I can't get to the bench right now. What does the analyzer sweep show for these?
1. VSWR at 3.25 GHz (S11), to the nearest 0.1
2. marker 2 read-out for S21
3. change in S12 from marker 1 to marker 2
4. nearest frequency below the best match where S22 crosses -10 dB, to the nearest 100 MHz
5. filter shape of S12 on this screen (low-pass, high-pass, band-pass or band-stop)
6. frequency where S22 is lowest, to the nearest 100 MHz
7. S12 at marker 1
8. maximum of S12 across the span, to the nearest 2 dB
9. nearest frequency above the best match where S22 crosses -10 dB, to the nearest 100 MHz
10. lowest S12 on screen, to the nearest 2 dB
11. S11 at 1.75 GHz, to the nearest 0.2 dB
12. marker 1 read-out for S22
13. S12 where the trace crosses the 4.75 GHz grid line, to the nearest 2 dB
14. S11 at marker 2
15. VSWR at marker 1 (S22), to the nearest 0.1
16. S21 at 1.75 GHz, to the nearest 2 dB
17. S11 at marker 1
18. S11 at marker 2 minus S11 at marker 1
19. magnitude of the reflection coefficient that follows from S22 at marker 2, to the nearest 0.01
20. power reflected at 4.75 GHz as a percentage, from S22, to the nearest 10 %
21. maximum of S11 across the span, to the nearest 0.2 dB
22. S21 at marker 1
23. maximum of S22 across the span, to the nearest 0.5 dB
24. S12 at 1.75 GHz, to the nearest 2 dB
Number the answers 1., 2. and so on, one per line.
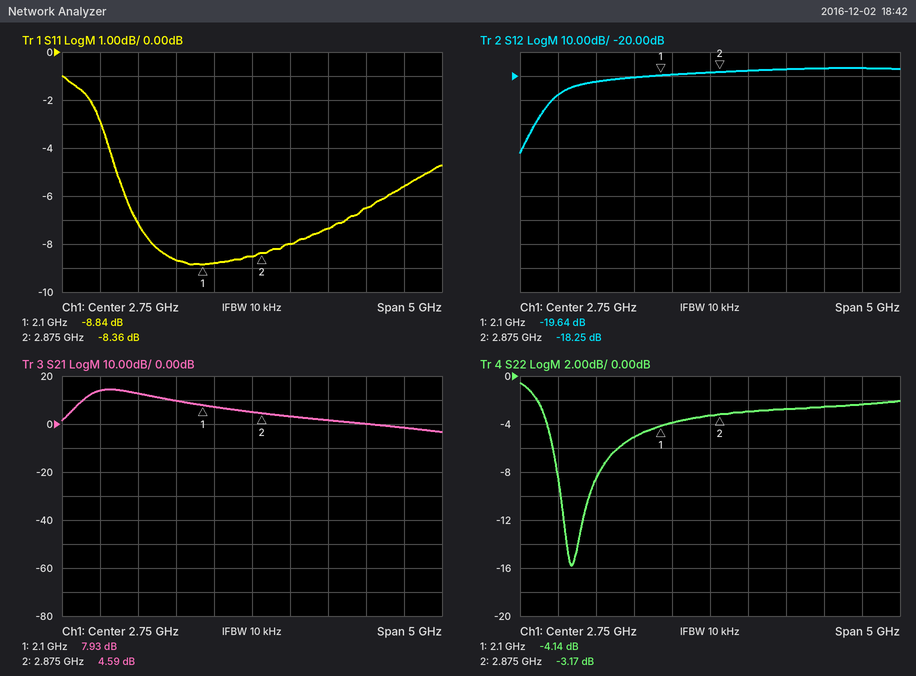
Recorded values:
1. 2.3
2. 4.59 dB
3. 1.39 dB
4. 800 MHz
5. high-pass
6. 900 MHz
7. -19.64 dB
8. -16 dB
9. 1.2 GHz
10. -52 dB
11. -8.6 dB
12. -4.14 dB
13. -16 dB
14. -8.36 dB
15. 4.3
16. 10 dB
17. -8.84 dB
18. 0.48 dB
19. 0.69
20. 60 %
21. -1.0 dB
22. 7.93 dB
23. -0.5 dB
24. -20 dB
